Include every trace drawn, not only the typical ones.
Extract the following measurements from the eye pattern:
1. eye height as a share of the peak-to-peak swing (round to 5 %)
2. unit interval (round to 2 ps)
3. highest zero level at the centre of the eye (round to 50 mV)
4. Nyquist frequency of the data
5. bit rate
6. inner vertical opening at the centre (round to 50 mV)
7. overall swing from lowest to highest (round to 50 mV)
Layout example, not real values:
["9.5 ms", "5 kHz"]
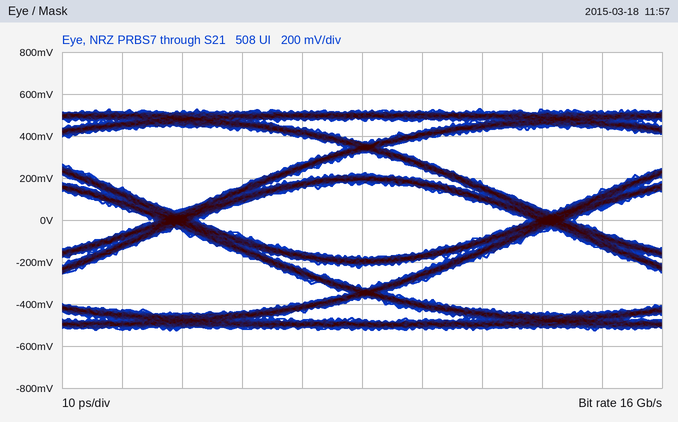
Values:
["35 %", "62 ps", "-200 mV", "8 GHz", "16 Gb/s", "350 mV", "1.05 V"]
